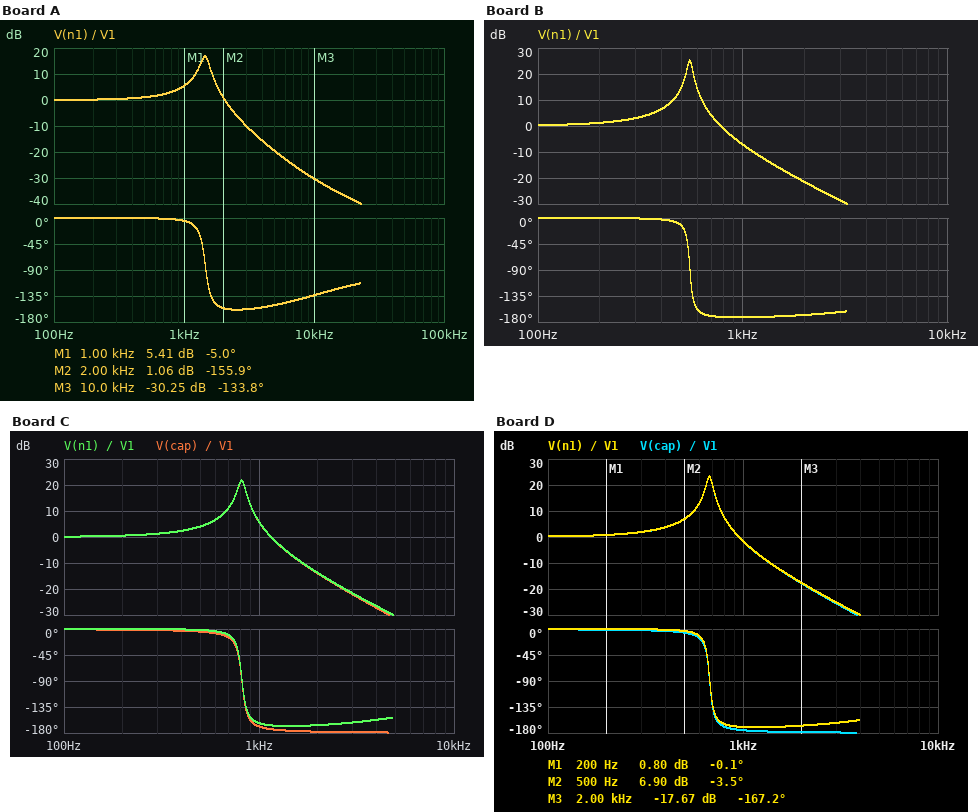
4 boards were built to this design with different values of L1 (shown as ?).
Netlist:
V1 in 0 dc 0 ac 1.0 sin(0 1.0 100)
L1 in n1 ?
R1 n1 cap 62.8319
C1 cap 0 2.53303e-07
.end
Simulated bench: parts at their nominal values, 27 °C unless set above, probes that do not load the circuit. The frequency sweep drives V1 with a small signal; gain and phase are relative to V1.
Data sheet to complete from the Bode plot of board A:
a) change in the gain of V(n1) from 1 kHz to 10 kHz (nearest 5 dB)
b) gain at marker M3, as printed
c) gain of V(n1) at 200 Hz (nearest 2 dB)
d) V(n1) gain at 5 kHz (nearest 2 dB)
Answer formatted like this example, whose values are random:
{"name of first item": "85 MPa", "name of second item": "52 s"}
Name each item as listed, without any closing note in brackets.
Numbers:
{"change in the gain of V(n1) from 1 kHz to 10 kHz": "-35 dB", "gain at marker M3, as printed": "-30.25 dB", "gain of V(n1) at 200 Hz": "0 dB", "V(n1) gain at 5 kHz": "-20 dB"}
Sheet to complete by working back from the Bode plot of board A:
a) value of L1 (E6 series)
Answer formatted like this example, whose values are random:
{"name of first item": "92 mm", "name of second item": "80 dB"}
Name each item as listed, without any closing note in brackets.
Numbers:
{"value of L1": "47 mH"}
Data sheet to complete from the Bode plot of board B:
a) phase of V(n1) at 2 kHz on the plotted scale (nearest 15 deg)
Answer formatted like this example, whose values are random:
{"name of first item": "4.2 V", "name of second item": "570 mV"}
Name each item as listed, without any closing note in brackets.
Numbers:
{"phase of V(n1) at 2 kHz on the plotted scale": "-165 deg"}
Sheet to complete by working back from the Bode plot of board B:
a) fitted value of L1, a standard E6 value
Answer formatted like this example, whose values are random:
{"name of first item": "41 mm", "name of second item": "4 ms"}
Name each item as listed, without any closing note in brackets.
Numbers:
{"fitted value of L1, a standard E6 value": "330 mH"}
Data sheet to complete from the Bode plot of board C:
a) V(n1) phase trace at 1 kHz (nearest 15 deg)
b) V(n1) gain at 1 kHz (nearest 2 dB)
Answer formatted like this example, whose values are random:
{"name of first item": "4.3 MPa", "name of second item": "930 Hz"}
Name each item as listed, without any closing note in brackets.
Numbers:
{"V(n1) phase trace at 1 kHz": "-165 deg", "V(n1) gain at 1 kHz": "6 dB"}
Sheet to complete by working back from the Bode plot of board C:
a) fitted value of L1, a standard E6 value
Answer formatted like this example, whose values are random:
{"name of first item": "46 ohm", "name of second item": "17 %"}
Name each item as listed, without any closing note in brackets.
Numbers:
{"fitted value of L1, a standard E6 value": "150 mH"}
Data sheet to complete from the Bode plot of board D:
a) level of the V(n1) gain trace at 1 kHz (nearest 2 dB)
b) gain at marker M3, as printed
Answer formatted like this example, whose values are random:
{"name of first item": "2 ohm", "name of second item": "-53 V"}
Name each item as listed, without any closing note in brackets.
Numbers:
{"level of the V(n1) gain trace at 1 kHz": "-2 dB", "gain at marker M3, as printed": "-17.67 dB"}
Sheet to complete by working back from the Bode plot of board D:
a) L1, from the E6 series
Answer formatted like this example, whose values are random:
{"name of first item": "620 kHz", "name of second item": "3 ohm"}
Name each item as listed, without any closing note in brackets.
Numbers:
{"L1, from the E6 series": "220 mH"}
